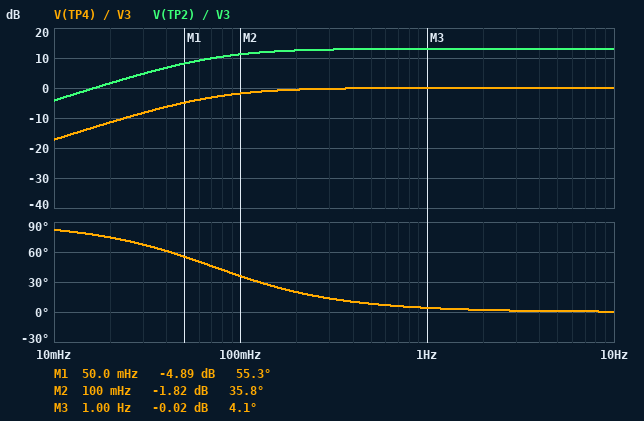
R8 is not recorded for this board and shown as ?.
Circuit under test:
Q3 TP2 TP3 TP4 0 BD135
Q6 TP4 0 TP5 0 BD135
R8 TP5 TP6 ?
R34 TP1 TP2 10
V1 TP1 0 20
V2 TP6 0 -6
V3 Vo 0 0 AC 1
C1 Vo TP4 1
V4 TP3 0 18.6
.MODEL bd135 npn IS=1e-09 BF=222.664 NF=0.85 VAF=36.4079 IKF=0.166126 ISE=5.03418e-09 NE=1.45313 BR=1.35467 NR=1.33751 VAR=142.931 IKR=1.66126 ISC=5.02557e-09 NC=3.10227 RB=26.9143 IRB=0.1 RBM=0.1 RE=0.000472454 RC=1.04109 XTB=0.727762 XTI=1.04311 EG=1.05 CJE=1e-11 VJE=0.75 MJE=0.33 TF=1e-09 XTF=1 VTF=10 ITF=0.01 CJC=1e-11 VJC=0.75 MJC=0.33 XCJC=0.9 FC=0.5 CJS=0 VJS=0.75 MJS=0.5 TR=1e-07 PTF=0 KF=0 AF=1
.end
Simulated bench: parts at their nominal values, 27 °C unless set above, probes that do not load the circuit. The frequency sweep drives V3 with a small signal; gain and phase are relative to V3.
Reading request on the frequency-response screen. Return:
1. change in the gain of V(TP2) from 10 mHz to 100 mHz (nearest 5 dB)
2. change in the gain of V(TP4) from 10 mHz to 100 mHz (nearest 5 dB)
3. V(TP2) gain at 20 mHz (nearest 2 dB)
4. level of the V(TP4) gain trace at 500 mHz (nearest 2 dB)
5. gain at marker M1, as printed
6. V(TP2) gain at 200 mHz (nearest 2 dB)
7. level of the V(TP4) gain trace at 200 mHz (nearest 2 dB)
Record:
15 dB
15 dB
2 dB
0 dB
-4.89 dB
12 dB
0 dB
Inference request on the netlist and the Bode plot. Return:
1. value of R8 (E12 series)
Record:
470 Ω
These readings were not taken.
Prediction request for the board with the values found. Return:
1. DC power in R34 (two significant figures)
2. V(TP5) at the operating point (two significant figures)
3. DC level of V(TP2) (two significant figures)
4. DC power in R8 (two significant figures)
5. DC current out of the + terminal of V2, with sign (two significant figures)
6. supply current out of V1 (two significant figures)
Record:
1.4 mW
-350 mV
20 V
68 mW
-12 mA
12 mA
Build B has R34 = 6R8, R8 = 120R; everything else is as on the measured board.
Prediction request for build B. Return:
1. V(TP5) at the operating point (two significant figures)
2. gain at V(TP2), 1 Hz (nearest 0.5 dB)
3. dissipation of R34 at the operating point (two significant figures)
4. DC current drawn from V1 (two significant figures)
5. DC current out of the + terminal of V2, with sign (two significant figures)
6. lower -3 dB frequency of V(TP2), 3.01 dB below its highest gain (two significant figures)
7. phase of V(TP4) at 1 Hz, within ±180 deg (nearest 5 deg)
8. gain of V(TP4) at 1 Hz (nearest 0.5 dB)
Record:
-390 mV
18.0 dB
14 mW
46 mA
-47 mA
190 mHz
10 deg
0 dB
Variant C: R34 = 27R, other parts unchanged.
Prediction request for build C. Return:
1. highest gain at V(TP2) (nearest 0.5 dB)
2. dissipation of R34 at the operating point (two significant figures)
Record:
21.5 dB
3.8 mW
